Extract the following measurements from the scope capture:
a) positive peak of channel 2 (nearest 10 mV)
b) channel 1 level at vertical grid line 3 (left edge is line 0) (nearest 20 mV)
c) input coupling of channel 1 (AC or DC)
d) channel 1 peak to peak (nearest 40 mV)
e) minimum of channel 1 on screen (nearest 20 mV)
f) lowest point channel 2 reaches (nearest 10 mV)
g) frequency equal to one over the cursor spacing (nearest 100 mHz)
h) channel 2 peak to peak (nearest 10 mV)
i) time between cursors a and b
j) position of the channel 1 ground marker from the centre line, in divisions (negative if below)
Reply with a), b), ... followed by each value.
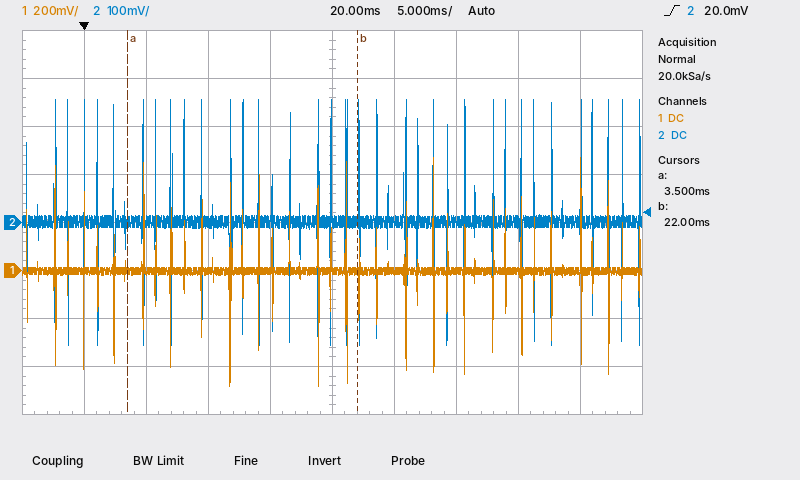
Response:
a) 260 mV
b) 0 mV
c) DC
d) 960 mV
e) -480 mV
f) -250 mV
g) 54.1 Hz
h) 510 mV
i) 18.5 ms
j) -1.0 div
